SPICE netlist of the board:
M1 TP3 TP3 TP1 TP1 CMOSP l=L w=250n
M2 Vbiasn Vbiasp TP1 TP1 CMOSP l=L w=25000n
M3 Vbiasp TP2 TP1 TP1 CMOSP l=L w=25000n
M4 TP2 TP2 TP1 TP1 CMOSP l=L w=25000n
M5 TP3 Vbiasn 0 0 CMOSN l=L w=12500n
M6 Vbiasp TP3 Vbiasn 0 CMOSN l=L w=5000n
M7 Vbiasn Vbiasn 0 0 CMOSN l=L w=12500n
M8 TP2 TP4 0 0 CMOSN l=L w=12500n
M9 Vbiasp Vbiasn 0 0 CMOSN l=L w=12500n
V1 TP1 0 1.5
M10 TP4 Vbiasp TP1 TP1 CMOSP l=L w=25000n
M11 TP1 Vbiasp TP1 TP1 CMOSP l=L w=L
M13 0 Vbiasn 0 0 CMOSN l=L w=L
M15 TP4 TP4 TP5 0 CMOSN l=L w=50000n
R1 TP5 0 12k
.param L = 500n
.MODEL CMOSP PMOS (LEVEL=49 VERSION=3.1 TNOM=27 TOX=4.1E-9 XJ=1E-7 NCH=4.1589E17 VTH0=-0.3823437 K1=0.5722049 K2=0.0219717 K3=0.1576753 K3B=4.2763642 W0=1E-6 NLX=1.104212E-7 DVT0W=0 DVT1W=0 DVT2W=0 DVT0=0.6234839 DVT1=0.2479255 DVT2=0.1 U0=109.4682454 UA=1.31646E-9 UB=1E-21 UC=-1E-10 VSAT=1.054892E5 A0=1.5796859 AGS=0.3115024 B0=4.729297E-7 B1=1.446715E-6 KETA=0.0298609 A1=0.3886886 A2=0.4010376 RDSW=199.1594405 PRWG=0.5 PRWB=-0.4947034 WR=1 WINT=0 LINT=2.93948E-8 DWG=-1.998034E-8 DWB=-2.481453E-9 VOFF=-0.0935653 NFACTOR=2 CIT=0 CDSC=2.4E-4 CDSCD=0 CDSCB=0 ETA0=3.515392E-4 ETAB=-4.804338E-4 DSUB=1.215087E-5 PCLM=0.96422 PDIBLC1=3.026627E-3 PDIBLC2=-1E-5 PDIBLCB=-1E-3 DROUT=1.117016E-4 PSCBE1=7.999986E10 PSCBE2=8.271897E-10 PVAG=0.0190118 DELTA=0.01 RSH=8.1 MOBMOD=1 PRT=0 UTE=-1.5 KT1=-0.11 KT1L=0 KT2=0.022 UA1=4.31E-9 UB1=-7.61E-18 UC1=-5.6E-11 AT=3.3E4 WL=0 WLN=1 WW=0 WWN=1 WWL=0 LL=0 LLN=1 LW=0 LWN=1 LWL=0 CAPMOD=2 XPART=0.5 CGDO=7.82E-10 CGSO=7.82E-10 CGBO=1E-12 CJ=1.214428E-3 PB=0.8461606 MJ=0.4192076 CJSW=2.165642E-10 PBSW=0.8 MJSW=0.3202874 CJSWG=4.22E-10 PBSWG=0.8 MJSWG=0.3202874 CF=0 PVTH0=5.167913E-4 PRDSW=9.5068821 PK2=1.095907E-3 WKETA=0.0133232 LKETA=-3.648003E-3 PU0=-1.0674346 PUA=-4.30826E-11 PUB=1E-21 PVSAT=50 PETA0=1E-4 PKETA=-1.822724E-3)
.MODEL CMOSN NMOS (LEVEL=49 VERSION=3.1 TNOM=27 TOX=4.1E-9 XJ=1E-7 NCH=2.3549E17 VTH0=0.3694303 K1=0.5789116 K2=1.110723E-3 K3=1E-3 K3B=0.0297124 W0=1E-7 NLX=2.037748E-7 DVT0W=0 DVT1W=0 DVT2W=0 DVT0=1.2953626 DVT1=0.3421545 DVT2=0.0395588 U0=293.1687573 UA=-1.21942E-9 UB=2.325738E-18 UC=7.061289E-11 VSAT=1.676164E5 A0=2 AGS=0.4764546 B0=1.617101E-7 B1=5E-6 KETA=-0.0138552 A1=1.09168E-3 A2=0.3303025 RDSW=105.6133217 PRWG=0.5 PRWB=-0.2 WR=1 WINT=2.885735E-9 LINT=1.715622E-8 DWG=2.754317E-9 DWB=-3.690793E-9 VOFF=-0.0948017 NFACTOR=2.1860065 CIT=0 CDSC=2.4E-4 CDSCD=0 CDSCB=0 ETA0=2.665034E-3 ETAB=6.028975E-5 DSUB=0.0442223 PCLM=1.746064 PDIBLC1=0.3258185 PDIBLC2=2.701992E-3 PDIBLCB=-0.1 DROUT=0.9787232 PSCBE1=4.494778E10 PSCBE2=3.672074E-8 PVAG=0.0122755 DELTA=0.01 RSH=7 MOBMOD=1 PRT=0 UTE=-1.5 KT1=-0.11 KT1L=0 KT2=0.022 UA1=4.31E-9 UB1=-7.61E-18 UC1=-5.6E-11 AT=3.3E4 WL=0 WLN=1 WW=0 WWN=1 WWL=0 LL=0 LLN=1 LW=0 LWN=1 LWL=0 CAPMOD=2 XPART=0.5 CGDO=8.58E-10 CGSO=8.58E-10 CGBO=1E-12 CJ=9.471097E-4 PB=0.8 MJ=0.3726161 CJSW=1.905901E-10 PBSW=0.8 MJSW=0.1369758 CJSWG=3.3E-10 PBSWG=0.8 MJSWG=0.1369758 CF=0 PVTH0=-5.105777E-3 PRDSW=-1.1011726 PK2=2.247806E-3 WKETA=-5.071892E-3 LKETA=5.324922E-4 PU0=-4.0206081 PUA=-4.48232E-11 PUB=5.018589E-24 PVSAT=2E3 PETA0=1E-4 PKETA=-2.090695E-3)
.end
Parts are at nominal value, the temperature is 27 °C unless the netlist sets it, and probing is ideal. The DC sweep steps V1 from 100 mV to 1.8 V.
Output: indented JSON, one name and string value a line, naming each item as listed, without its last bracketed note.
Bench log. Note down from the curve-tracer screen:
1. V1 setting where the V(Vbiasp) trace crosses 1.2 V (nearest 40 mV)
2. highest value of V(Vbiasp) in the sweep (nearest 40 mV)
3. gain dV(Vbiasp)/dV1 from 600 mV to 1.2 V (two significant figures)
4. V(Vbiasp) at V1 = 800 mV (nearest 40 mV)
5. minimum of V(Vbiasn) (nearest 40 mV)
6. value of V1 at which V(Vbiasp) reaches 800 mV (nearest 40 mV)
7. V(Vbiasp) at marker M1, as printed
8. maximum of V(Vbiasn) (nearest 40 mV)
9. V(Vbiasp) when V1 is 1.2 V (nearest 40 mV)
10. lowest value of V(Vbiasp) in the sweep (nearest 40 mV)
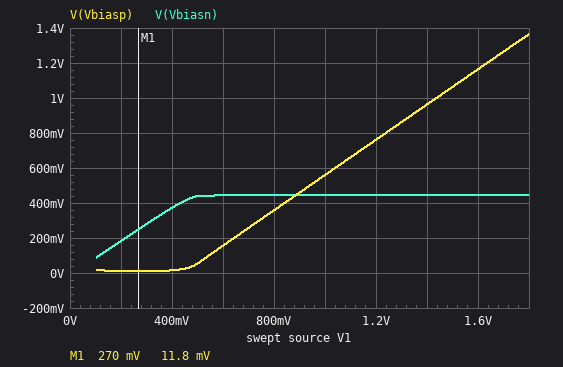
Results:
{
  "V1 setting where the V(Vbiasp) trace crosses 1.2 V": "1.64 V",
  "highest value of V(Vbiasp) in the sweep": "1.36 V",
  "gain dV(Vbiasp)/dV1 from 600 mV to 1.2 V": "1.0 V/V",
  "V(Vbiasp) at V1 = 800 mV": "360 mV",
  "minimum of V(Vbiasn)": "80 mV",
  "value of V1 at which V(Vbiasp) reaches 800 mV": "1.24 V",
  "V(Vbiasp) at marker M1, as printed": "11.8 mV",
  "maximum of V(Vbiasn)": "440 mV",
  "V(Vbiasp) when V1 is 1.2 V": "760 mV",
  "lowest value of V(Vbiasp) in the sweep": "0 V"
}
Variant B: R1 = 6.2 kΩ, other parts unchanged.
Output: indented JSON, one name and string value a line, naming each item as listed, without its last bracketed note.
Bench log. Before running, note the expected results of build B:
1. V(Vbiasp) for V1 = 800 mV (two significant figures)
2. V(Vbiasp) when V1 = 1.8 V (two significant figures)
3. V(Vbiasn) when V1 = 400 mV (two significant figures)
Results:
{
  "V(Vbiasp) for V1 = 800 mV": "320 mV",
  "V(Vbiasp) when V1 = 1.8 V": "1.3 V",
  "V(Vbiasn) when V1 = 400 mV": "370 mV"
}
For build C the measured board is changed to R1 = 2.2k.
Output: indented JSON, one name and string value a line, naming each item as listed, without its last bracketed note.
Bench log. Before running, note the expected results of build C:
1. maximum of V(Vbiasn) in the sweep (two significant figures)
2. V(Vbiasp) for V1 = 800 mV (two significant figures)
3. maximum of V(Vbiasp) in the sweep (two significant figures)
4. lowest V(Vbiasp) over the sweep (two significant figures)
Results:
{
  "maximum of V(Vbiasn) in the sweep": "530 mV",
  "V(Vbiasp) for V1 = 800 mV": "250 mV",
  "maximum of V(Vbiasp) in the sweep": "1.3 V",
  "lowest V(Vbiasp) over the sweep": "11 mV"
}
